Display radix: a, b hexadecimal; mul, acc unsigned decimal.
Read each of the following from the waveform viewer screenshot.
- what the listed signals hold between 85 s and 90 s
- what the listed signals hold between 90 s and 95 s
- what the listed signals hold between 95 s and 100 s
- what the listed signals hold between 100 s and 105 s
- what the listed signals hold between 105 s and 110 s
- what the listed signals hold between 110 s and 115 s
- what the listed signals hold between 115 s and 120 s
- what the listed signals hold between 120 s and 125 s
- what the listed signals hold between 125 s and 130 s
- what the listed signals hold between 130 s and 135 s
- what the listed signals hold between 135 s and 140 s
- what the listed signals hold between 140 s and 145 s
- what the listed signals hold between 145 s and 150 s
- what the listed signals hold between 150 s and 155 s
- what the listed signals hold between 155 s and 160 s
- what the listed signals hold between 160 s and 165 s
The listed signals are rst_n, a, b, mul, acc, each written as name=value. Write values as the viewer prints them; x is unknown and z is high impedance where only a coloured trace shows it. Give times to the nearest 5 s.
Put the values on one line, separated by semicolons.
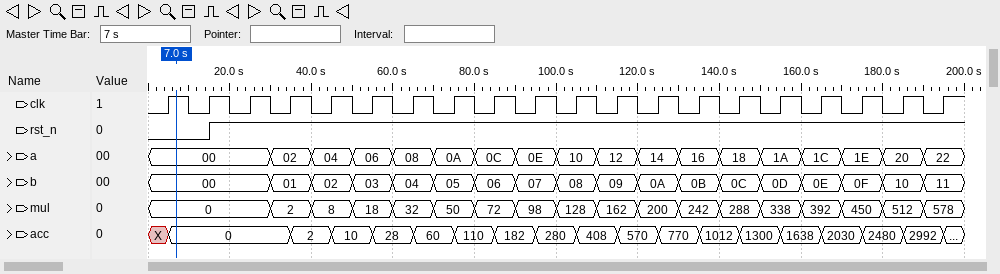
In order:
rst_n=1, a=0C, b=06, mul=72, acc=182; rst_n=1, a=0E, b=07, mul=98, acc=182; rst_n=1, a=0E, b=07, mul=98, acc=280; rst_n=1, a=10, b=08, mul=128, acc=280; rst_n=1, a=10, b=08, mul=128, acc=408; rst_n=1, a=12, b=09, mul=162, acc=408; rst_n=1, a=12, b=09, mul=162, acc=570; rst_n=1, a=14, b=0A, mul=200, acc=570; rst_n=1, a=14, b=0A, mul=200, acc=770; rst_n=1, a=16, b=0B, mul=242, acc=770; rst_n=1, a=16, b=0B, mul=242, acc=1012; rst_n=1, a=18, b=0C, mul=288, acc=1012; rst_n=1, a=18, b=0C, mul=288, acc=1300; rst_n=1, a=1A, b=0D, mul=338, acc=1300; rst_n=1, a=1A, b=0D, mul=338, acc=1638; rst_n=1, a=1C, b=0E, mul=392, acc=1638
